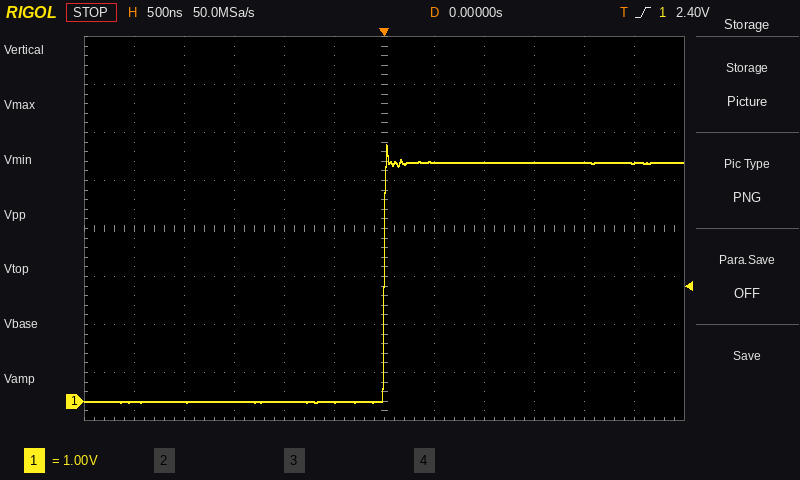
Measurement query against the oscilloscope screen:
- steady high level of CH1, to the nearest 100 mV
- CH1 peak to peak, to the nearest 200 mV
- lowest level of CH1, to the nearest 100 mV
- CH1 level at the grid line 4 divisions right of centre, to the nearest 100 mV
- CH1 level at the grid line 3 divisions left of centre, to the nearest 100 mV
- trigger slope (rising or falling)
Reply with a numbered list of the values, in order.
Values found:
1. 5.0 V
2. 5.4 V
3. 0.0 V
4. 5.0 V
5. 0.0 V
6. rising
